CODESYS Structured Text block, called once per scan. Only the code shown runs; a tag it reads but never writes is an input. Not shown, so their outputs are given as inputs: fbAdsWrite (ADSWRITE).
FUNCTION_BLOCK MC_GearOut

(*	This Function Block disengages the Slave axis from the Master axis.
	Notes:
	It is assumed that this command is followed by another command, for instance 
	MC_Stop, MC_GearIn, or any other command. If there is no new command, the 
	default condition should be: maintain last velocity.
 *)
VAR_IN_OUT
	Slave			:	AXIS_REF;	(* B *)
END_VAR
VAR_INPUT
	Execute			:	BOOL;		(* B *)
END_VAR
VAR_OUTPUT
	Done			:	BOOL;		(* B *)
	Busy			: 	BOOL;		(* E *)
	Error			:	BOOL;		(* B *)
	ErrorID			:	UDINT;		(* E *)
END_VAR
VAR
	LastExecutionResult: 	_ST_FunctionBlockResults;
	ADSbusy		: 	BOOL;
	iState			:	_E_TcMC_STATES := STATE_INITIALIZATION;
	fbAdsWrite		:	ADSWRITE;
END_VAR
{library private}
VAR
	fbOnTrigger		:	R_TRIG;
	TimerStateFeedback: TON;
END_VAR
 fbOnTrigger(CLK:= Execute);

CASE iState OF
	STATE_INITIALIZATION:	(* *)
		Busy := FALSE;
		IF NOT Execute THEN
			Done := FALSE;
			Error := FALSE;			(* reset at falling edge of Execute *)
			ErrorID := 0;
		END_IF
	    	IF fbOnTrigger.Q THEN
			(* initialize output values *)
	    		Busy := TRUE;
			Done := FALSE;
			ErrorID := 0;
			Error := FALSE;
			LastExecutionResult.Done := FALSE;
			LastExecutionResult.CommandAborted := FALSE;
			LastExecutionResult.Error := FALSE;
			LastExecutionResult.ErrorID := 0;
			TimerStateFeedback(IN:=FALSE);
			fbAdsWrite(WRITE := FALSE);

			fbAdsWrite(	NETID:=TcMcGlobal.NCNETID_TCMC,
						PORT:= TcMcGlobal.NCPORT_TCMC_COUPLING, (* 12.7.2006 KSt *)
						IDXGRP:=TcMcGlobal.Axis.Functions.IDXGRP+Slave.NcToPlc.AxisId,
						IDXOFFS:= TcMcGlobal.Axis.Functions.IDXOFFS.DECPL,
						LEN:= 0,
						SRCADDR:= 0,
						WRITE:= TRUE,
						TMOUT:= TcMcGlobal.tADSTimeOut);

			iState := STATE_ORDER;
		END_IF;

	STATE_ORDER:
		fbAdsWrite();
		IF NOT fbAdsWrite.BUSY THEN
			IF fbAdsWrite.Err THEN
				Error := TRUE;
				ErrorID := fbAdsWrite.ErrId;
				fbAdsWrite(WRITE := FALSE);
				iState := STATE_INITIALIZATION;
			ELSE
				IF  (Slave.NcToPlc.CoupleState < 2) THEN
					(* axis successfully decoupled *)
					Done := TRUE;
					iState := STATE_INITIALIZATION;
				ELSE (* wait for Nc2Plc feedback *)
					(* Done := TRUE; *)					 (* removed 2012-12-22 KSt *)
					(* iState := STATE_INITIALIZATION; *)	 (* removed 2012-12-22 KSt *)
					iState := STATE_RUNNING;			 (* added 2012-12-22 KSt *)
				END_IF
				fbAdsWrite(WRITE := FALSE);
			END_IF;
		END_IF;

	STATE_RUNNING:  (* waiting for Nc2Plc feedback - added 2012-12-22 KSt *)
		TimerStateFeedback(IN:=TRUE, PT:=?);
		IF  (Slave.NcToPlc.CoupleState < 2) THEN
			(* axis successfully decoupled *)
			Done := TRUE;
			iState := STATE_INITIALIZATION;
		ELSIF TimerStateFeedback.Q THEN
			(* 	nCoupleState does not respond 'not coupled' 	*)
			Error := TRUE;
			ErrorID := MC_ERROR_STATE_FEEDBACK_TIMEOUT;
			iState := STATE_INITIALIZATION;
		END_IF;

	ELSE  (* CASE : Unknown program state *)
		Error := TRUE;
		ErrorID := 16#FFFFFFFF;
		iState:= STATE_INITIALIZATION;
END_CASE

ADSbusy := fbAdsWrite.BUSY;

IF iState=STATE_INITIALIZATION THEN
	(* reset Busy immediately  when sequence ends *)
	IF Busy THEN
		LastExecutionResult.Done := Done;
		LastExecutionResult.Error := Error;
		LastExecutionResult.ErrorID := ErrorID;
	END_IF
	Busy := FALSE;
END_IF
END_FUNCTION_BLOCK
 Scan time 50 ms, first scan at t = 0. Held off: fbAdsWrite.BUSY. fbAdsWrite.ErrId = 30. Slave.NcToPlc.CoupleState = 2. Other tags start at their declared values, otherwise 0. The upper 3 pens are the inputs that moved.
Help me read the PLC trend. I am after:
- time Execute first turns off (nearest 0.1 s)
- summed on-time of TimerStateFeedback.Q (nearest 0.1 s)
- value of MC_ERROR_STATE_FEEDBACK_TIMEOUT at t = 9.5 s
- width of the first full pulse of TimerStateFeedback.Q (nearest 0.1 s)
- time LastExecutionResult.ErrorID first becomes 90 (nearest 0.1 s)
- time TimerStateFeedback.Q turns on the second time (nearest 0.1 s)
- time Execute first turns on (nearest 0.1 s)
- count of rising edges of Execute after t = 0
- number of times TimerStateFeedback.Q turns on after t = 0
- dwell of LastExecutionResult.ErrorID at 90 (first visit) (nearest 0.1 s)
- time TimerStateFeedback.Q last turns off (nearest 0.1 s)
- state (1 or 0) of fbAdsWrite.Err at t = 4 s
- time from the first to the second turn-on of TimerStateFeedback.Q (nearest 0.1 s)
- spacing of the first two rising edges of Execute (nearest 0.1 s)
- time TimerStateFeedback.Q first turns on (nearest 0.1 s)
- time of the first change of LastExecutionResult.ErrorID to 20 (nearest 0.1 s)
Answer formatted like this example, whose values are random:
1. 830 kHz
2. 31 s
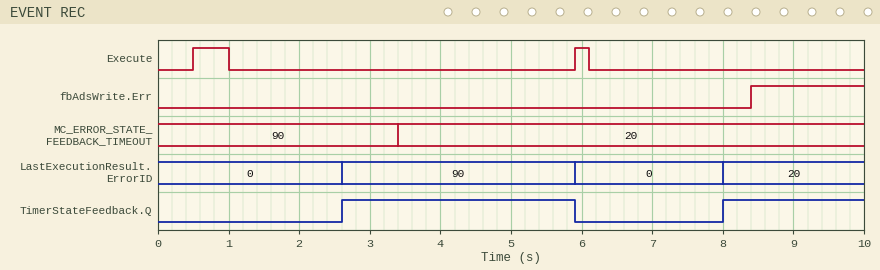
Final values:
1. 1.0 s
2. 5.3 s
3. 20
4. 3.3 s
5. 2.6 s
6. 8.0 s
7. 0.5 s
8. 2
9. 2
10. 3.3 s
11. 5.9 s
12. 0
13. 5.4 s
14. 5.4 s
15. 2.6 s
16. 8.0 s
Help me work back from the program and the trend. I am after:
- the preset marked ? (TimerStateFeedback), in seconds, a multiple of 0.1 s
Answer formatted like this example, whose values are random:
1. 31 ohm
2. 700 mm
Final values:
1. 2.0 s
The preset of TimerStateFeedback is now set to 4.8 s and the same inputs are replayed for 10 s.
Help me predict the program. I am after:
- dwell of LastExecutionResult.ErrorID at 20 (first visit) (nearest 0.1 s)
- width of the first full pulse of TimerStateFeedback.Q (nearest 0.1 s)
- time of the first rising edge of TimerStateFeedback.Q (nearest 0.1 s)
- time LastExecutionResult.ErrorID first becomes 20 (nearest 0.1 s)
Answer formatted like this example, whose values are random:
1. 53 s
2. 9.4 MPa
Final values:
1. 0.5 s
2. 0.5 s
3. 5.4 s
4. 5.4 s
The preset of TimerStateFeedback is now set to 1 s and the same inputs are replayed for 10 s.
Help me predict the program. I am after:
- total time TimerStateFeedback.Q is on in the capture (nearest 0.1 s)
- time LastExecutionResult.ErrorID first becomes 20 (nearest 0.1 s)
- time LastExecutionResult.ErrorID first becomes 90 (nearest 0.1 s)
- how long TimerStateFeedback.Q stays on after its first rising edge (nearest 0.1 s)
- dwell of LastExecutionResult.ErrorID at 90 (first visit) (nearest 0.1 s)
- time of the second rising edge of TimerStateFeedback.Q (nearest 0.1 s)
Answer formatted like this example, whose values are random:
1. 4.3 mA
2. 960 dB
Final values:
1. 7.3 s
2. 7.0 s
3. 1.6 s
4. 4.3 s
5. 4.3 s
6. 7.0 s
